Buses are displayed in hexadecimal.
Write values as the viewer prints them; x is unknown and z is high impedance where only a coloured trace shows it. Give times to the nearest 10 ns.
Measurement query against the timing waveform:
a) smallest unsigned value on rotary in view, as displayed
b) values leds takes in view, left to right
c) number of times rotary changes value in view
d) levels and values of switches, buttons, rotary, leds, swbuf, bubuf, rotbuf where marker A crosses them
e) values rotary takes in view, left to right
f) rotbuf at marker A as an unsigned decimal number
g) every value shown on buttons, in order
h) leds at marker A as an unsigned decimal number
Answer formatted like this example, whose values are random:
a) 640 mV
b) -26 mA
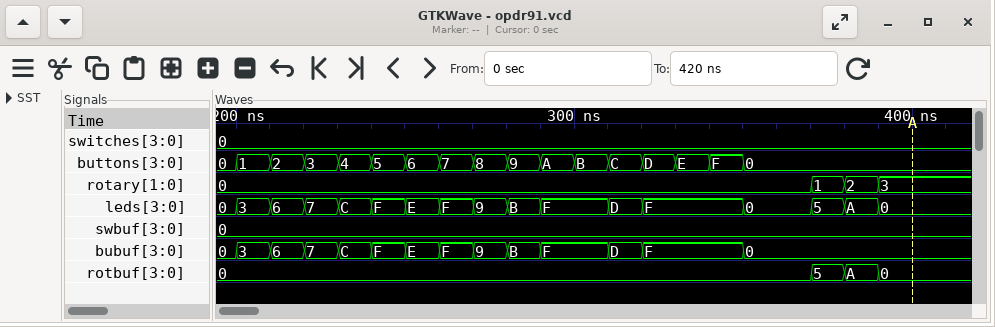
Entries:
a) 0
b) 0, 3, 6, 7, C, F, E, F, 9, B, F, D, F, 0, 5, A, 0
c) 3
d) switches=0, buttons=0, rotary=3, leds=0, swbuf=0, bubuf=0, rotbuf=0
e) 0, 1, 2, 3
f) 0
g) 0, 1, 2, 3, 4, 5, 6, 7, 8, 9, A, B, C, D, E, F, 0
h) 0
